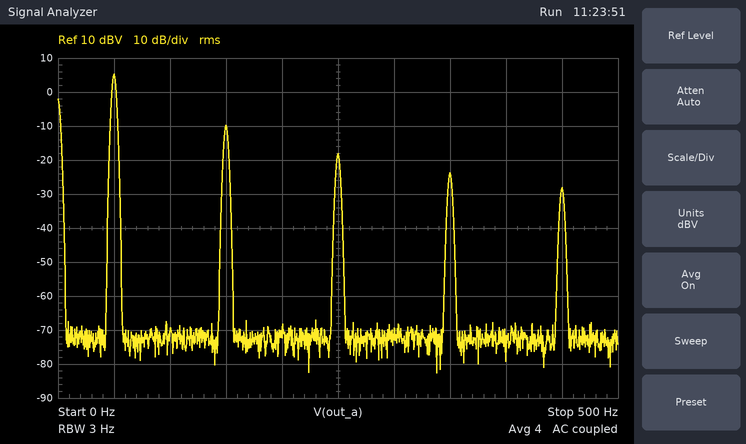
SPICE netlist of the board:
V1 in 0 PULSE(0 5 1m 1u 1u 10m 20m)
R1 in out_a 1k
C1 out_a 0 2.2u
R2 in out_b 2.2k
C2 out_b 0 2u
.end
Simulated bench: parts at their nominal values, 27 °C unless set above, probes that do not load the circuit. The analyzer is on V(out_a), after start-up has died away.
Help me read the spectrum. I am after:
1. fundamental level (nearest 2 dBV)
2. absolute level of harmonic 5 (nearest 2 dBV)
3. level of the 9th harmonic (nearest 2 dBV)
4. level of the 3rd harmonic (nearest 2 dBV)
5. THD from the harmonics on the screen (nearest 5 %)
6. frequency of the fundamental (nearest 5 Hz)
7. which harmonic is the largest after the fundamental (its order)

6 dBV
-18 dBV
-28 dBV
-10 dBV
20 %
50 Hz
3
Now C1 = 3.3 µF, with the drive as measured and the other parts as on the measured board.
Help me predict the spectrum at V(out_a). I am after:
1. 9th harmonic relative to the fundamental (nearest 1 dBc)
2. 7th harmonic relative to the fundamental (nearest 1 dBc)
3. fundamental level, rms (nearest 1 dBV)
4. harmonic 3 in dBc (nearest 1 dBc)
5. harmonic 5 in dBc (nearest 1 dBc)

-35 dBc
-31 dBc
4 dBV
-17 dBc
-25 dBc
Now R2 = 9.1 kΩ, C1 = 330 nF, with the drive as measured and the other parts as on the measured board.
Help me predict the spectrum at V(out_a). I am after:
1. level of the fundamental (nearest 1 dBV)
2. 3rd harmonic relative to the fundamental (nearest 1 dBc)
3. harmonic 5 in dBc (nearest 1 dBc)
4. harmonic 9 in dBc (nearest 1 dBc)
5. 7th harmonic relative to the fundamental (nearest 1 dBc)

7 dBV
-10 dBc
-15 dBc
-22 dBc
-19 dBc
